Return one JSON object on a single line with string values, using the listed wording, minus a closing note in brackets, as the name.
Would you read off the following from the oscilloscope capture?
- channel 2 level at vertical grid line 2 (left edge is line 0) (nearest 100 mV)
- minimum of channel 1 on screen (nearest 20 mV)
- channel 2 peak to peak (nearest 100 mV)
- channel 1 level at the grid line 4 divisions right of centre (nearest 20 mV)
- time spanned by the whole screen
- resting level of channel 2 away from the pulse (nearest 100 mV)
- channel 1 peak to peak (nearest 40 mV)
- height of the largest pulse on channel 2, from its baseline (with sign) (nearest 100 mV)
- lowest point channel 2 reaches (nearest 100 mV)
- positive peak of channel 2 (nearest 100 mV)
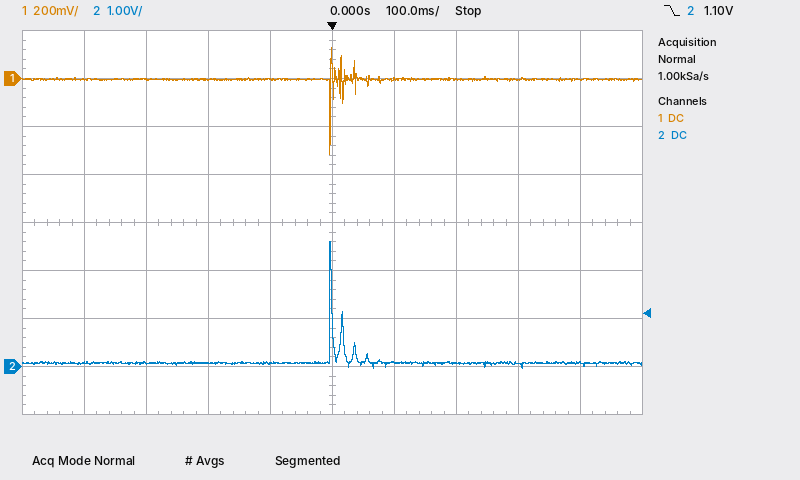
{"channel 2 level at vertical grid line 2 (left edge is line 0)": "100 mV", "minimum of channel 1 on screen": "-320 mV", "channel 2 peak to peak": "2.6 V", "channel 1 level at the grid line 4 divisions right of centre": "0 mV", "time spanned by the whole screen": "1 s", "resting level of channel 2 away from the pulse": "100 mV", "channel 1 peak to peak": "440 mV", "height of the largest pulse on channel 2, from its baseline (with sign)": "+2.5 V", "lowest point channel 2 reaches": "0.0 V", "positive peak of channel 2": "2.6 V"}
